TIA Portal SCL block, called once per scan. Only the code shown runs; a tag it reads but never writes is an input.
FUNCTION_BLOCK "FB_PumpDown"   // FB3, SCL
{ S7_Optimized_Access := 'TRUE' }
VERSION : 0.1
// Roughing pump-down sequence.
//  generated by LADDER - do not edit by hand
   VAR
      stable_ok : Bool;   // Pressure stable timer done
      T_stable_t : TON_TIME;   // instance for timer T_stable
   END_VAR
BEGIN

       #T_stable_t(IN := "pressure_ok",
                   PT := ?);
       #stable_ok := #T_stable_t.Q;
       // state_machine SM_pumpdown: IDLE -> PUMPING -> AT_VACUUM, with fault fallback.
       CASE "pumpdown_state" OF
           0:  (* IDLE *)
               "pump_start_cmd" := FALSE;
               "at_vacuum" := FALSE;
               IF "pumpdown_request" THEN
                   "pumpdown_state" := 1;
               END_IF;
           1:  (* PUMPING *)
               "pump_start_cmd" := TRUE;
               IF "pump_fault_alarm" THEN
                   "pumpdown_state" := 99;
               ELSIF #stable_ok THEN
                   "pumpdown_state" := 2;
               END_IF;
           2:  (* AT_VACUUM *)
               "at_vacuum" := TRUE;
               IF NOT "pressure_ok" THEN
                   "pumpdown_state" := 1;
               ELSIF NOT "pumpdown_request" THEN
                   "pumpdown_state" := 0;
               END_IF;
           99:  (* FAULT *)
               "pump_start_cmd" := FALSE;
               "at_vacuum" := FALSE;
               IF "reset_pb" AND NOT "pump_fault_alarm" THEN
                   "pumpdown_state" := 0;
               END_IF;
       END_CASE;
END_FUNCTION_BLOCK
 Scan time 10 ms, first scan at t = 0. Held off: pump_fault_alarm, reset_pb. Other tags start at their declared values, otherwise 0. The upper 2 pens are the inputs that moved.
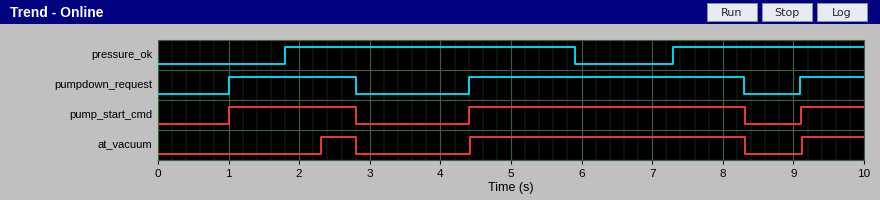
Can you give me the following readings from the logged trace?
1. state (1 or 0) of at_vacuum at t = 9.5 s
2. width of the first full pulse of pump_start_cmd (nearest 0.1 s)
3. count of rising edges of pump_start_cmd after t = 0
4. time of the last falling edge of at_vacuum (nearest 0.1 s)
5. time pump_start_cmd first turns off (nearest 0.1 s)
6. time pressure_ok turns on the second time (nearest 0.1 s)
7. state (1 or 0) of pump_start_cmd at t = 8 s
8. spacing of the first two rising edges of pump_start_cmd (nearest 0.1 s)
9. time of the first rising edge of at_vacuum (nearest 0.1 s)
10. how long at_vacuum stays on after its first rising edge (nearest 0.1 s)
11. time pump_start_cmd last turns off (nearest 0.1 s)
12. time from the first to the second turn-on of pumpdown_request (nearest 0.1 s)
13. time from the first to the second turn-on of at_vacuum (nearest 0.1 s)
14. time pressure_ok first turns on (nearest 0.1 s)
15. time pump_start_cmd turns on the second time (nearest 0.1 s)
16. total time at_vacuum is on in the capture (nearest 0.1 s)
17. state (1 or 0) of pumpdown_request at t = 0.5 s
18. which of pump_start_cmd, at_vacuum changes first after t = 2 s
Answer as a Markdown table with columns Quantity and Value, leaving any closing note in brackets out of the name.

| Quantity | Value |
|---|---|
| state (1 or 0) of at_vacuum at t = 9.5 s | 1 |
| width of the first full pulse of pump_start_cmd | 1.8 s |
| count of rising edges of pump_start_cmd after t = 0 | 3 |
| time of the last falling edge of at_vacuum | 8.3 s |
| time pump_start_cmd first turns off | 2.8 s |
| time pressure_ok turns on the second time | 7.3 s |
| state (1 or 0) of pump_start_cmd at t = 8 s | 1 |
| spacing of the first two rising edges of pump_start_cmd | 3.4 s |
| time of the first rising edge of at_vacuum | 2.3 s |
| how long at_vacuum stays on after its first rising edge | 0.5 s |
| time pump_start_cmd last turns off | 8.3 s |
| time from the first to the second turn-on of pumpdown_request | 3.4 s |
| time from the first to the second turn-on of at_vacuum | 2.1 s |
| time pressure_ok first turns on | 1.8 s |
| time pump_start_cmd turns on the second time | 4.4 s |
| total time at_vacuum is on in the capture | 5.3 s |
| state (1 or 0) of pumpdown_request at t = 0.5 s | 0 |
| which of pump_start_cmd, at_vacuum changes first after t = 2 s | at_vacuum |
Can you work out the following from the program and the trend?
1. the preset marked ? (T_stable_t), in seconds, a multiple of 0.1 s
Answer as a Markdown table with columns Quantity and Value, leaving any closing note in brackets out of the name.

| Quantity | Value |
|---|---|
| the preset marked ? (T_stable_t), in seconds, a multiple of 0.1 s | 0.5 s |
